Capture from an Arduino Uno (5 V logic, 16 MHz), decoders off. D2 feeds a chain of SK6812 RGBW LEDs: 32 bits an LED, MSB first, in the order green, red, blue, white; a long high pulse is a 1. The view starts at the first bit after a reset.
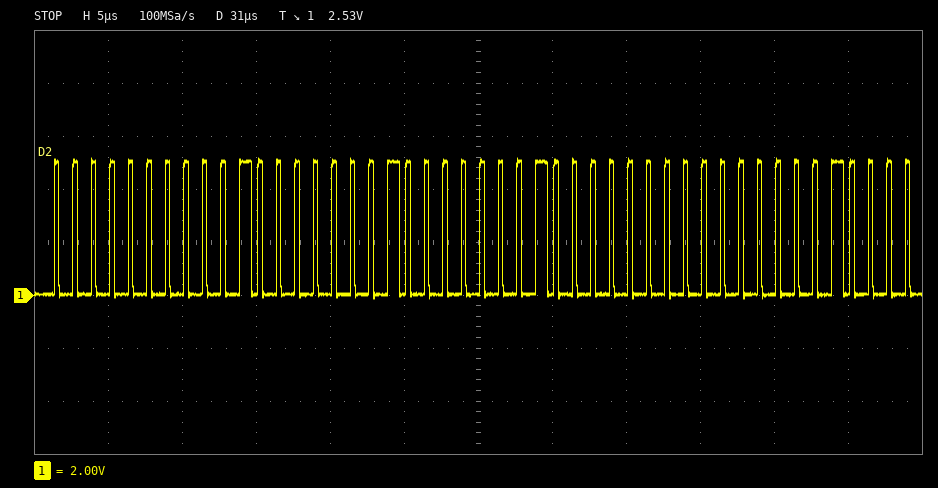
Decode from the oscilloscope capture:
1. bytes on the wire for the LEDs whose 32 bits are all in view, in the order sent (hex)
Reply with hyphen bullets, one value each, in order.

- 00 20 20 20
